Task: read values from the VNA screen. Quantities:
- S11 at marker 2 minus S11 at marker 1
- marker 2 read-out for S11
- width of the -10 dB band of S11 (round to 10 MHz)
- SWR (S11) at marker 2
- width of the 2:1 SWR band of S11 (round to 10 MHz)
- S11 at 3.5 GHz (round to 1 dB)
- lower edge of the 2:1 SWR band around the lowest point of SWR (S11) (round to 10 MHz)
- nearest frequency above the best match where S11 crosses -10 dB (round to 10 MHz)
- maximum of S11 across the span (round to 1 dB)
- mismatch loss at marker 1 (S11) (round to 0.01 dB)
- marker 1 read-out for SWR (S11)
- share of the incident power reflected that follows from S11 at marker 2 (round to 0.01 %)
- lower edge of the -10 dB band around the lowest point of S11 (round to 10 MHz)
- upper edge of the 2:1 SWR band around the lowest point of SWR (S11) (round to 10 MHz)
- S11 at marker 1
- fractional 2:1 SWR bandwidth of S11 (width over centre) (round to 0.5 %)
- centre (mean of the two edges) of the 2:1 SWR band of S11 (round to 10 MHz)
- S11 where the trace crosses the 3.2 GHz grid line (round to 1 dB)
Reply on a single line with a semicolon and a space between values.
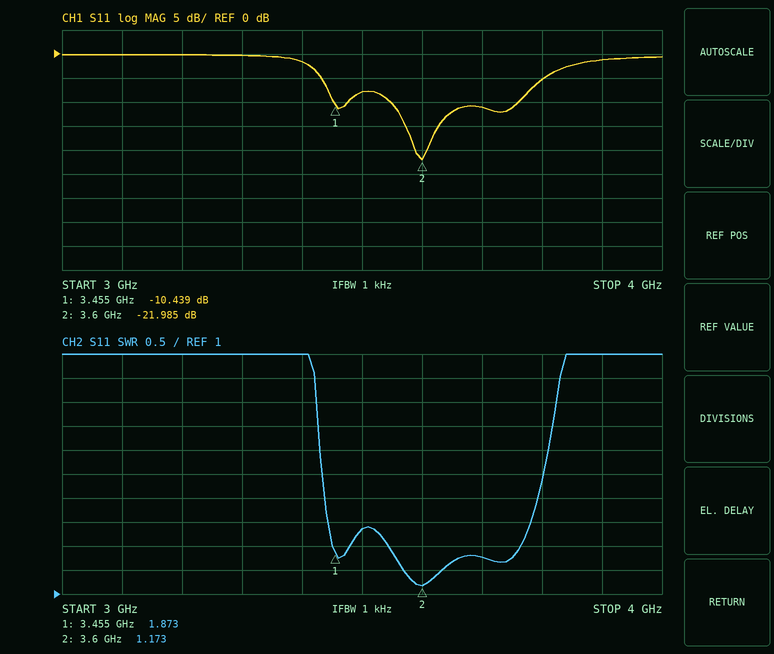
-11.546 dB; -21.985 dB; 210 MHz; 1.173; 220 MHz; -8 dB; 3.54 GHz; 3.76 GHz; 0 dB; 0.41 dB; 1.873; 0.63 %; 3.55 GHz; 3.76 GHz; -10.439 dB; 6.0 %; 3.65 GHz; 0 dB
